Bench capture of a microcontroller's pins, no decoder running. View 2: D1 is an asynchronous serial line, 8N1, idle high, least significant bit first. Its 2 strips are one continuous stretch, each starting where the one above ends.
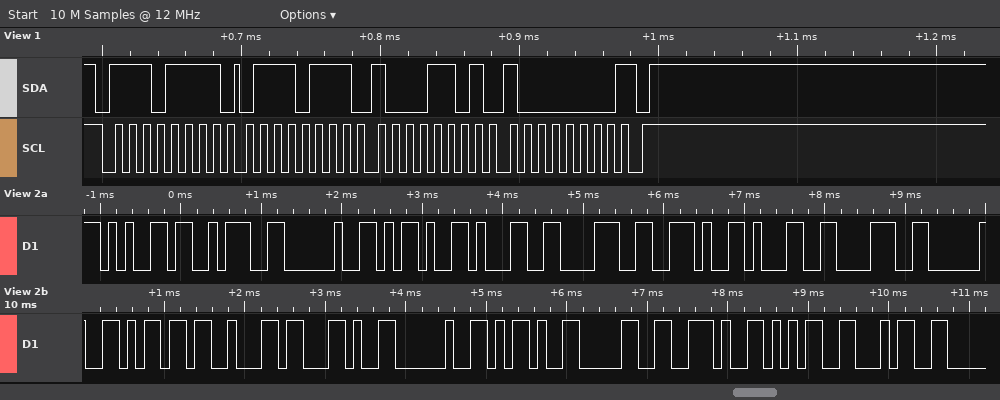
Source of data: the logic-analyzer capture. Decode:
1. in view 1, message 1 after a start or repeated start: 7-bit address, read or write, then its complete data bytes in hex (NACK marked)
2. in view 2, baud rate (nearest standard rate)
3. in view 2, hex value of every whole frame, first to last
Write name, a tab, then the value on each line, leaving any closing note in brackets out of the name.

in view 1, message 1 after a start or repeated start: 7-bit address, read or write, then its complete data bytes in hex	0x77 read: 77 8D 80 NACK
in view 2, baud rate	9600 baud
in view 2, hex value of every whole frame, first to last	65 3A 20 2D 31 38 2E 31 38 20 6D 62 2C 20 2D 30 2E 35 34
